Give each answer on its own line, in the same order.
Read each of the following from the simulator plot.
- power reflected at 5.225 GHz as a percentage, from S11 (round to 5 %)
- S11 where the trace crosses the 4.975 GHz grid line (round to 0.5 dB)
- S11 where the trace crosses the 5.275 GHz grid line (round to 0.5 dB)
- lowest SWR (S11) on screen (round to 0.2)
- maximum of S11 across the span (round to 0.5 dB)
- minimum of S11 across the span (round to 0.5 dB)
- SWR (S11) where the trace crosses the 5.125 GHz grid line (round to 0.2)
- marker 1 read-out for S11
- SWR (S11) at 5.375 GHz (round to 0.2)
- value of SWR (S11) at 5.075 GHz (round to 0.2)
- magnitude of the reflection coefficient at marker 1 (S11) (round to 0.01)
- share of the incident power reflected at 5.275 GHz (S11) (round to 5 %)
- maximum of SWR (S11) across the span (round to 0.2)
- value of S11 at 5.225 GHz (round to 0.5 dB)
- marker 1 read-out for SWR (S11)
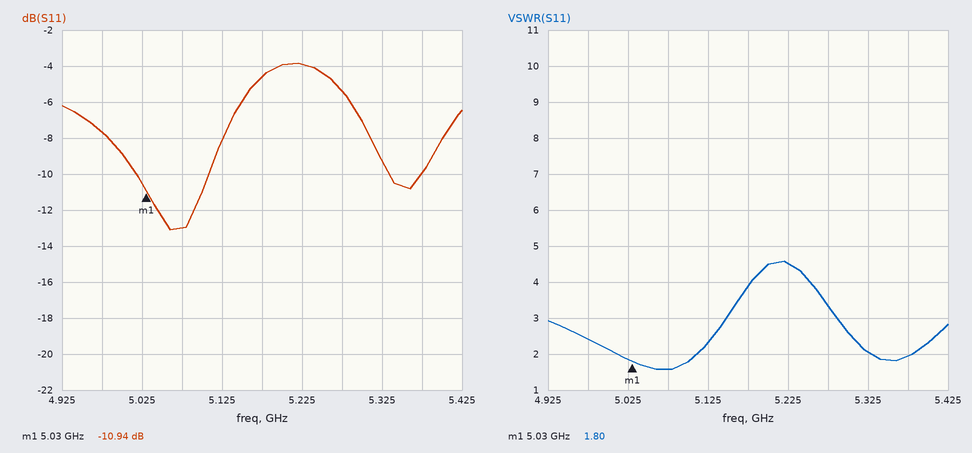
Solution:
40 %
-7.5 dB
-5.5 dB
1.6
-4.0 dB
-13.0 dB
2.4
-10.94 dB
2.0
1.6
0.28
30 %
4.6
-4.0 dB
1.80
